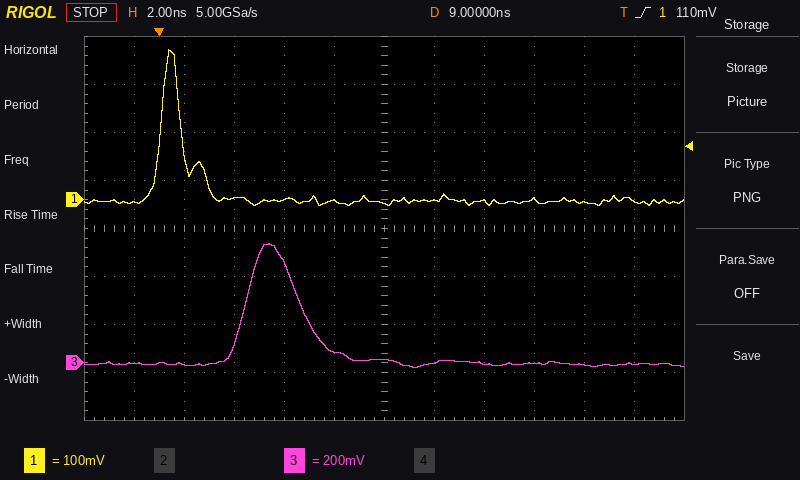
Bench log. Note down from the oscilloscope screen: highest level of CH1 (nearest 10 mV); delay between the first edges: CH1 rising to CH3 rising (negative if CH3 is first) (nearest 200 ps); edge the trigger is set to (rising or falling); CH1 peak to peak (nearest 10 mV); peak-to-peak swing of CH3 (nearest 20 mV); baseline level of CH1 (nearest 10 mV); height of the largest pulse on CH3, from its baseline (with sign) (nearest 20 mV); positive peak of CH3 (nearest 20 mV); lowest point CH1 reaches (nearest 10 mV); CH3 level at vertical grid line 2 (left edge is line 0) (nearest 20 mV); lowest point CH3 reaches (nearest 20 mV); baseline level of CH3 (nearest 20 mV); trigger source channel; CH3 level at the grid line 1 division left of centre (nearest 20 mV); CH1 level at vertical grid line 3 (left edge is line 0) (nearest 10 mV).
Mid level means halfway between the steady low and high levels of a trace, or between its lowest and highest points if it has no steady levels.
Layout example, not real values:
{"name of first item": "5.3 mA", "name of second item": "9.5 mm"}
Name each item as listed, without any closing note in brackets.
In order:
{"highest level of CH1": "310 mV", "delay between the first edges: CH1 rising to CH3 rising (negative if CH3 is first)": "+3.4 ns", "edge the trigger is set to": "rising", "CH1 peak to peak": "320 mV", "peak-to-peak swing of CH3": "520 mV", "baseline level of CH1": "0 mV", "height of the largest pulse on CH3, from its baseline (with sign)": "+500 mV", "positive peak of CH3": "500 mV", "lowest point CH1 reaches": "-10 mV", "CH3 level at vertical grid line 2 (left edge is line 0)": "0 mV", "lowest point CH3 reaches": "-20 mV", "baseline level of CH3": "0 mV", "trigger source channel": "CH1", "CH3 level at the grid line 1 division left of centre": "40 mV", "CH1 level at vertical grid line 3 (left edge is line 0)": "0 mV"}
